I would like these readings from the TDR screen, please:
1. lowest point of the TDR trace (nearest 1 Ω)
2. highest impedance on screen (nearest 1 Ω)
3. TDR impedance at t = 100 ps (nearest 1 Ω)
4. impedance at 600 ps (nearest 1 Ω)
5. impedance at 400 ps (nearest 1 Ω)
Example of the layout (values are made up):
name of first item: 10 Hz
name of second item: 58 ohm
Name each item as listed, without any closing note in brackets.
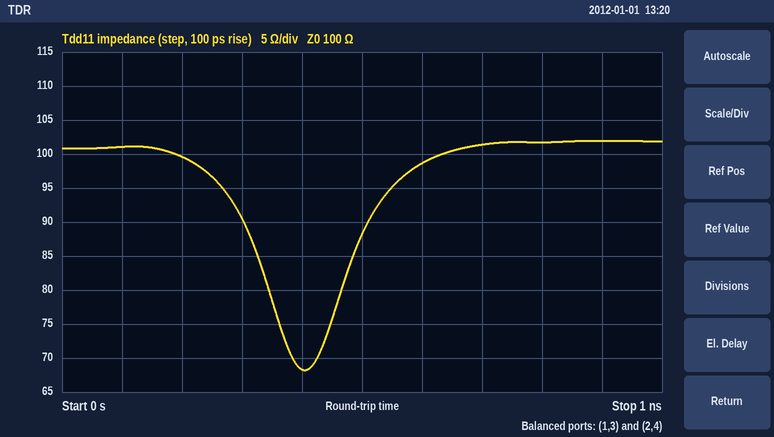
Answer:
lowest point of the TDR trace: 68 Ω
highest impedance on screen: 102 Ω
TDR impedance at t = 100 ps: 101 Ω
impedance at 600 ps: 99 Ω
impedance at 400 ps: 68 Ω
